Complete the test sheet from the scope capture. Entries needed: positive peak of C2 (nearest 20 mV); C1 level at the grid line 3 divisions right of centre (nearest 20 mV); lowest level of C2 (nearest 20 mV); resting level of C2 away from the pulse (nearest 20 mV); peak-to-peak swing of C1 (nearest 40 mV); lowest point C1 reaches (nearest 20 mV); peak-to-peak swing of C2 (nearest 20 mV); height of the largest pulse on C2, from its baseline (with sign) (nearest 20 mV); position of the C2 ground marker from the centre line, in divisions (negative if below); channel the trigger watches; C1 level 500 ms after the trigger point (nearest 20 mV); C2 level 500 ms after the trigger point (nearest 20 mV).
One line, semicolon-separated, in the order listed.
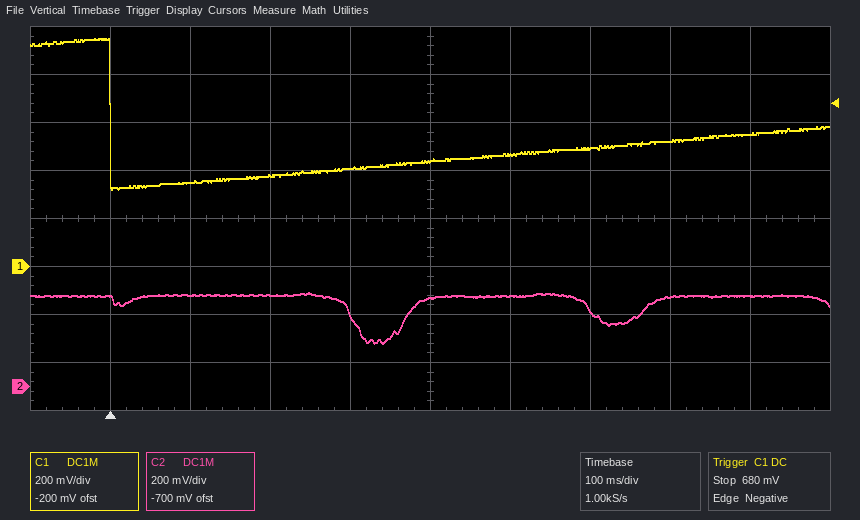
400 mV; 520 mV; 180 mV; 380 mV; 640 mV; 320 mV; 220 mV; -200 mV; -3.5 div; C1; 460 mV; 380 mV
